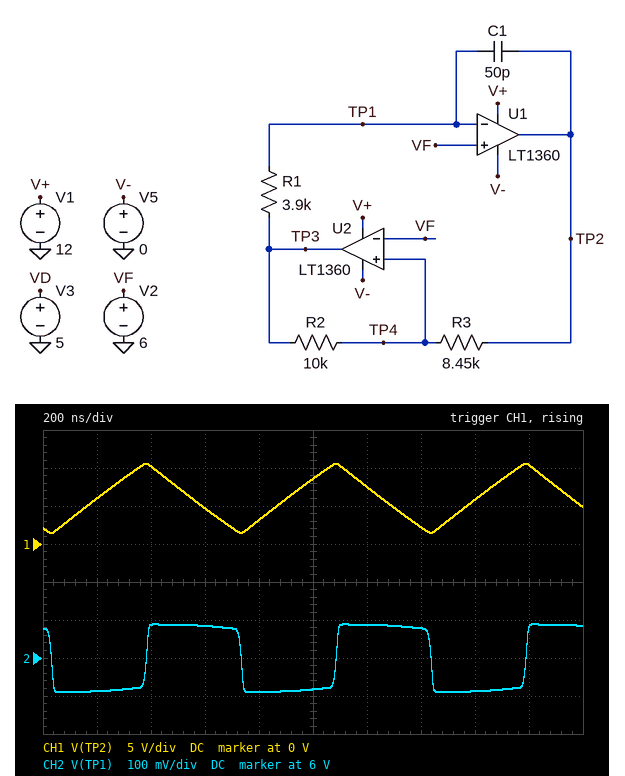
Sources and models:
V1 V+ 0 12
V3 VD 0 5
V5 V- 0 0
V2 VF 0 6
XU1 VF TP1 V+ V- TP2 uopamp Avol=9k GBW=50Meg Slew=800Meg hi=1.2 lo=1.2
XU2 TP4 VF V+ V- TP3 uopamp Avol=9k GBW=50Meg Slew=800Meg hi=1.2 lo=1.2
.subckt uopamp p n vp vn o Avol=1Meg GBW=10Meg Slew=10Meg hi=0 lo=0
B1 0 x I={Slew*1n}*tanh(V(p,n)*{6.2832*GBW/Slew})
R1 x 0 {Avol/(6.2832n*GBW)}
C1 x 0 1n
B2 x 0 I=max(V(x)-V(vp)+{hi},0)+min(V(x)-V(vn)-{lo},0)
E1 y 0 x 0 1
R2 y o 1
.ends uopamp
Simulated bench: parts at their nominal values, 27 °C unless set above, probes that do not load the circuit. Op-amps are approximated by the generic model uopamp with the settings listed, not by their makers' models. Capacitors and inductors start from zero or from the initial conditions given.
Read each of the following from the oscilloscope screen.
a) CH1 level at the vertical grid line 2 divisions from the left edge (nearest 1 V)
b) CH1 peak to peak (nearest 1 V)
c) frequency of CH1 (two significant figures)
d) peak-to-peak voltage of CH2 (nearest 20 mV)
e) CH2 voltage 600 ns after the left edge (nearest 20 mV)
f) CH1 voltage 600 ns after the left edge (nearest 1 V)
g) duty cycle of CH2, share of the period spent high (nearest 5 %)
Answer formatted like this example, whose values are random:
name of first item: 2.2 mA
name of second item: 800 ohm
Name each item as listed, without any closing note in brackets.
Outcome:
CH1 level at the vertical grid line 2 divisions from the left edge: 10 V
CH1 peak to peak: 9 V
frequency of CH1: 1.4 MHz
peak-to-peak voltage of CH2: 180 mV
CH2 voltage 600 ns after the left edge: 6.08 V
CH1 voltage 600 ns after the left edge: 5 V
duty cycle of CH2, share of the period spent high: 50 %
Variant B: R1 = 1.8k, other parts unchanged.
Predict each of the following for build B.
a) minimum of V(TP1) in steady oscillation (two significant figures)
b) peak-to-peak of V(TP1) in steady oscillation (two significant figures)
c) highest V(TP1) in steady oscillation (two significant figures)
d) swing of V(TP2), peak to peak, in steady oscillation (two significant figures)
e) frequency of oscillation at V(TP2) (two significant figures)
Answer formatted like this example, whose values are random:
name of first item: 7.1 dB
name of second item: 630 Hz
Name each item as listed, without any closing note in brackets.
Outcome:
minimum of V(TP1) in steady oscillation: 5.8 V
peak-to-peak of V(TP1) in steady oscillation: 380 mV
highest V(TP1) in steady oscillation: 6.2 V
swing of V(TP2), peak to peak, in steady oscillation: 9.7 V
frequency of oscillation at V(TP2): 2.7 MHz
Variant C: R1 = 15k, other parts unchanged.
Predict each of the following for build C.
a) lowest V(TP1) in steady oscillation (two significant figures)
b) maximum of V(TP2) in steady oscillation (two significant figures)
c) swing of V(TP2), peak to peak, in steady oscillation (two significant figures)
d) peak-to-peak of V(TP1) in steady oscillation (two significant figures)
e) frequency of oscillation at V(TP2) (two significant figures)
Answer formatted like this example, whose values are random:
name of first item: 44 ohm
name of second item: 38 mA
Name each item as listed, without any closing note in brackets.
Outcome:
lowest V(TP1) in steady oscillation: 6.0 V
maximum of V(TP2) in steady oscillation: 10 V
swing of V(TP2), peak to peak, in steady oscillation: 8.5 V
peak-to-peak of V(TP1) in steady oscillation: 46 mV
frequency of oscillation at V(TP2): 410 kHz
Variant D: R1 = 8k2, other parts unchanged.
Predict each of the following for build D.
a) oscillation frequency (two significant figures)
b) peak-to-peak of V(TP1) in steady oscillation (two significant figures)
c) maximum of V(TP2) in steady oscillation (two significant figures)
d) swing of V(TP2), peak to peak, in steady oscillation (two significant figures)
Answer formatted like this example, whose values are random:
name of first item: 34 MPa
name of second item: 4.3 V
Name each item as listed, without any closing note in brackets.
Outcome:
oscillation frequency: 730 kHz
peak-to-peak of V(TP1) in steady oscillation: 85 mV
maximum of V(TP2) in steady oscillation: 10 V
swing of V(TP2), peak to peak, in steady oscillation: 8.7 V
